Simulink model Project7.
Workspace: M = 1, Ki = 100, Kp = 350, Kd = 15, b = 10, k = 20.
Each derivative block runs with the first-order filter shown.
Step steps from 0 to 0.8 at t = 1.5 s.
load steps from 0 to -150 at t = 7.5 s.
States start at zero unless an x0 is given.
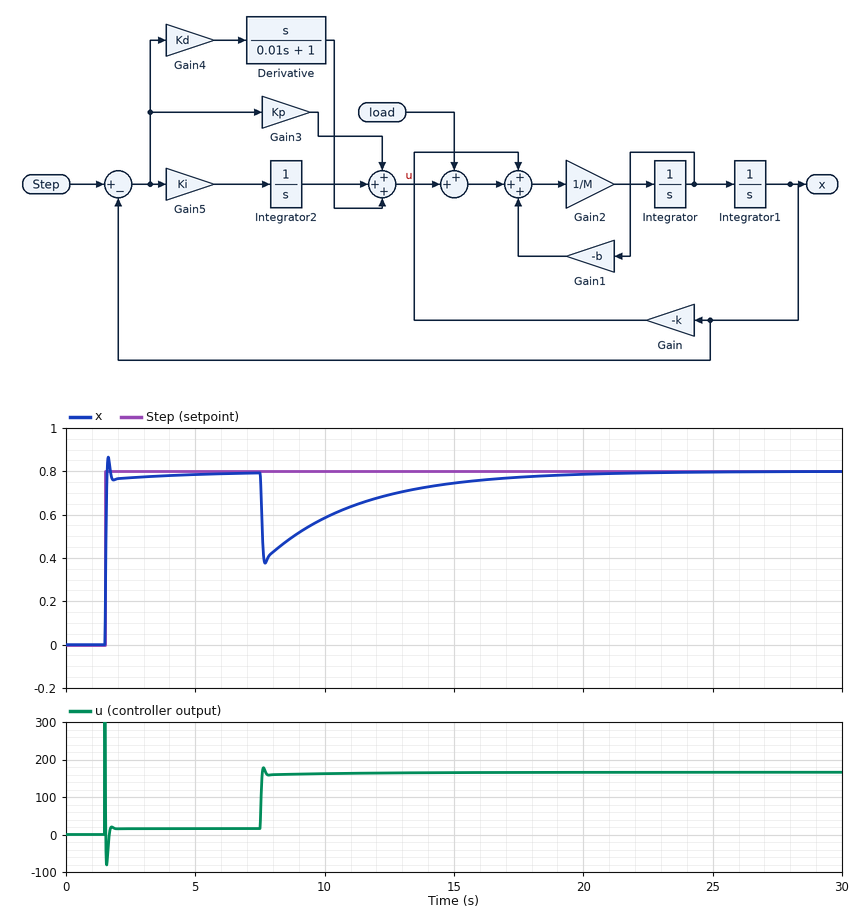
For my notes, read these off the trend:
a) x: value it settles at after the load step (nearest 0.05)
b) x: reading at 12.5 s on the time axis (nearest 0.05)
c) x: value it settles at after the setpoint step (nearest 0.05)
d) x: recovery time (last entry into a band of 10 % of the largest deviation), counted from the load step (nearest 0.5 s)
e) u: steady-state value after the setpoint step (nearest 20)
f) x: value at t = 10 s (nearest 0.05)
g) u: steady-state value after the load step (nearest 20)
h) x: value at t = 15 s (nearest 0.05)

0.80
0.70
0.80
8.5 s
20
0.60
160
0.75
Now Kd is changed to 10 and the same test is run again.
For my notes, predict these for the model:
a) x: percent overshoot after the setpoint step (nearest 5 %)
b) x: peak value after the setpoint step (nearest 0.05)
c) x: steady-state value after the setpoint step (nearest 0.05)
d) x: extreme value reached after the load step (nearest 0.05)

15 %
0.90
0.80
0.35
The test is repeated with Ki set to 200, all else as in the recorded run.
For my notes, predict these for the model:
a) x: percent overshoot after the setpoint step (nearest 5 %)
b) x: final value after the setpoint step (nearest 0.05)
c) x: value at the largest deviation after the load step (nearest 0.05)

10 %
0.80
0.40
